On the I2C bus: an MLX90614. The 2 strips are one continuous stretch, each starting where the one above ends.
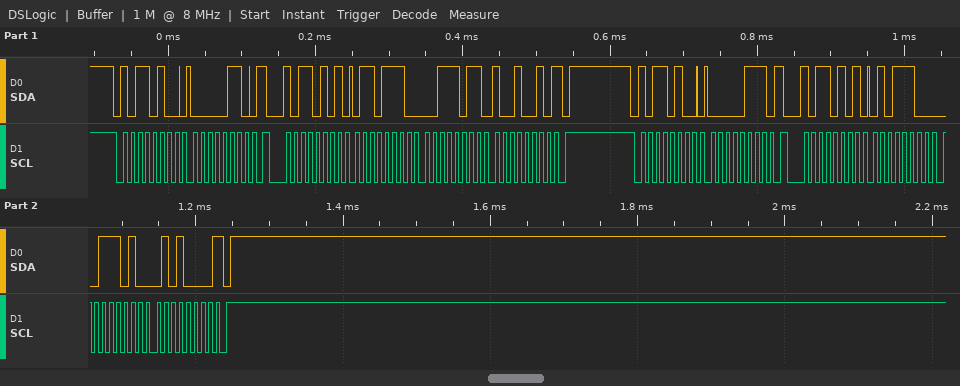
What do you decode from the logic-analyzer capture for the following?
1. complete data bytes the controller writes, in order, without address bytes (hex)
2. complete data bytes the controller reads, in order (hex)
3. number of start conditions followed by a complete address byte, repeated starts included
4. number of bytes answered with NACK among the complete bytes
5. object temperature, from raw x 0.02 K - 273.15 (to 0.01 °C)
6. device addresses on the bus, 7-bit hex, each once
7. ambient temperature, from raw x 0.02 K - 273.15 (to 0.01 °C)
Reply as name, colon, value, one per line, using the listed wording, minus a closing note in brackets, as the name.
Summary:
complete data bytes the controller writes, in order, without address bytes: 06 07
complete data bytes the controller reads, in order: 6E 3B 92 5C 3A 50
number of start conditions followed by a complete address byte, repeated starts included: 4
number of bytes answered with NACK among the complete bytes: 2
object temperature, from raw x 0.02 K - 273.15: 25.65 °C
device addresses on the bus, 7-bit hex, each once: 0x5A
ambient temperature, from raw x 0.02 K - 273.15: 31.13 °C
